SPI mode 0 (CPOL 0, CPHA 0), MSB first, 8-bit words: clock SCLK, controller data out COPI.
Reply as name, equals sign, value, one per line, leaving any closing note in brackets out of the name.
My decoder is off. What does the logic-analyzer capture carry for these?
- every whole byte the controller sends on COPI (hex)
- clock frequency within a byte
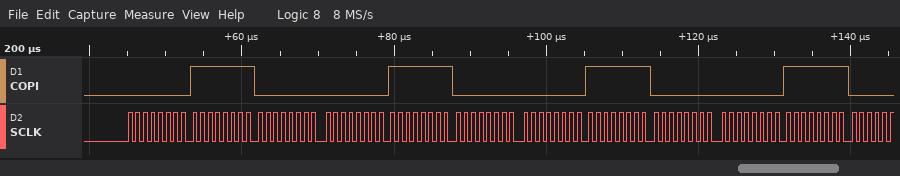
every whole byte the controller sends on COPI = 00 FF 00 00 FF 00 00 FF 00 00 FF
clock frequency within a byte = 1 MHz
